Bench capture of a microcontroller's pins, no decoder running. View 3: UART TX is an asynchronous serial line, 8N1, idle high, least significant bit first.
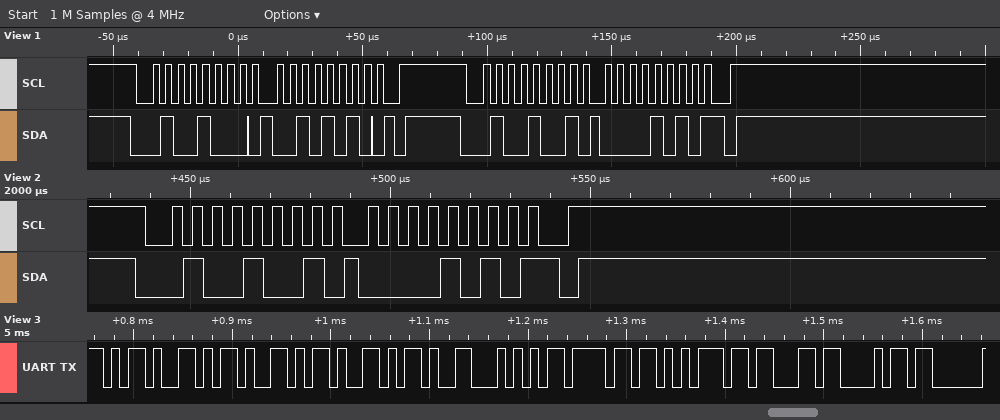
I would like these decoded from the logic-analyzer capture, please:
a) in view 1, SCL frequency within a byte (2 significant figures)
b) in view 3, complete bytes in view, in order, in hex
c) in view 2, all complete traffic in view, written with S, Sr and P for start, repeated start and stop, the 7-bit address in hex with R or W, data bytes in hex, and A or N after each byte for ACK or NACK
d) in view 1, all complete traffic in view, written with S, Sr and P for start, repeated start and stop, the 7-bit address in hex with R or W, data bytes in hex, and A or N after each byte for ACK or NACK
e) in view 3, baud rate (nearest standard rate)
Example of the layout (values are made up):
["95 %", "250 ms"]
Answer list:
["200 kHz", "2D 2D 2D 2D 54 6F 75 63 68", "S 24R A 0A N P", "S 24W A 2A A P S 24R A 0A N P", "115200 baud"]
